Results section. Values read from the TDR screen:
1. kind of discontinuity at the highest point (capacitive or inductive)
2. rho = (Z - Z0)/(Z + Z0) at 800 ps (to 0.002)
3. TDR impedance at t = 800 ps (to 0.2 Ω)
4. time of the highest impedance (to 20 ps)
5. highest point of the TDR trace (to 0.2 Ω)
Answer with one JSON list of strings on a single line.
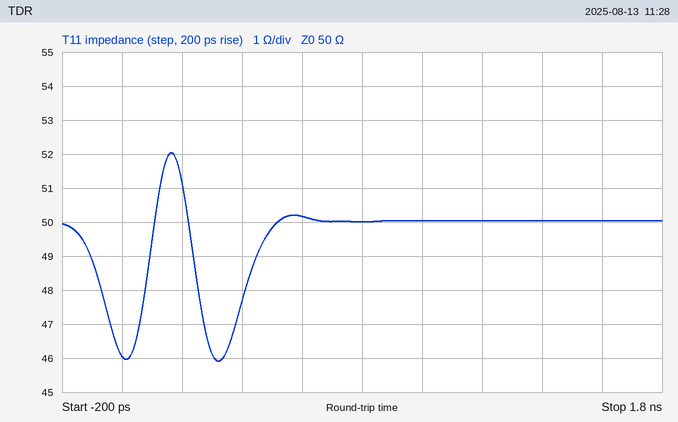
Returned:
["inductive", "0.000", "50.0 Ω", "160 ps", "52.0 Ω"]
